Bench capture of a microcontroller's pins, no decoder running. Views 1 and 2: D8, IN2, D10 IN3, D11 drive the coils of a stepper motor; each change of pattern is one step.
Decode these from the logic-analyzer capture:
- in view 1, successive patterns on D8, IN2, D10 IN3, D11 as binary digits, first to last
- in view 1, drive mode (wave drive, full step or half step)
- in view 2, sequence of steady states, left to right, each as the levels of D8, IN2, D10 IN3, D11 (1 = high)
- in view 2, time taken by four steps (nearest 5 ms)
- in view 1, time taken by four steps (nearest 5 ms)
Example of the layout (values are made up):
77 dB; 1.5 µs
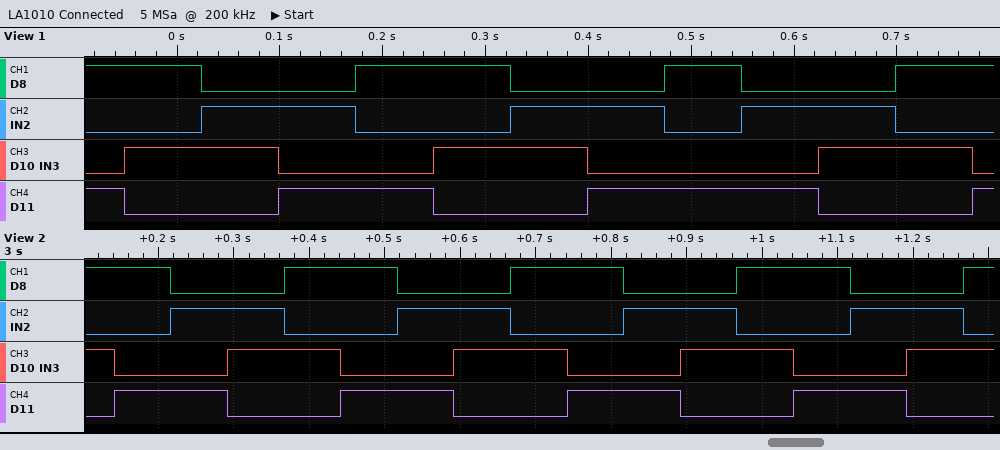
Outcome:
1001 1010 0110 0101 1001 1010 0110 0101 1001 0101 0110 1010 1001; full step; 1010 1001 0101 0110 1010 1001 0101 0110 1010 1001 0101 0110 1010 1001 0101 0110 1010; 300 ms; 300 ms
